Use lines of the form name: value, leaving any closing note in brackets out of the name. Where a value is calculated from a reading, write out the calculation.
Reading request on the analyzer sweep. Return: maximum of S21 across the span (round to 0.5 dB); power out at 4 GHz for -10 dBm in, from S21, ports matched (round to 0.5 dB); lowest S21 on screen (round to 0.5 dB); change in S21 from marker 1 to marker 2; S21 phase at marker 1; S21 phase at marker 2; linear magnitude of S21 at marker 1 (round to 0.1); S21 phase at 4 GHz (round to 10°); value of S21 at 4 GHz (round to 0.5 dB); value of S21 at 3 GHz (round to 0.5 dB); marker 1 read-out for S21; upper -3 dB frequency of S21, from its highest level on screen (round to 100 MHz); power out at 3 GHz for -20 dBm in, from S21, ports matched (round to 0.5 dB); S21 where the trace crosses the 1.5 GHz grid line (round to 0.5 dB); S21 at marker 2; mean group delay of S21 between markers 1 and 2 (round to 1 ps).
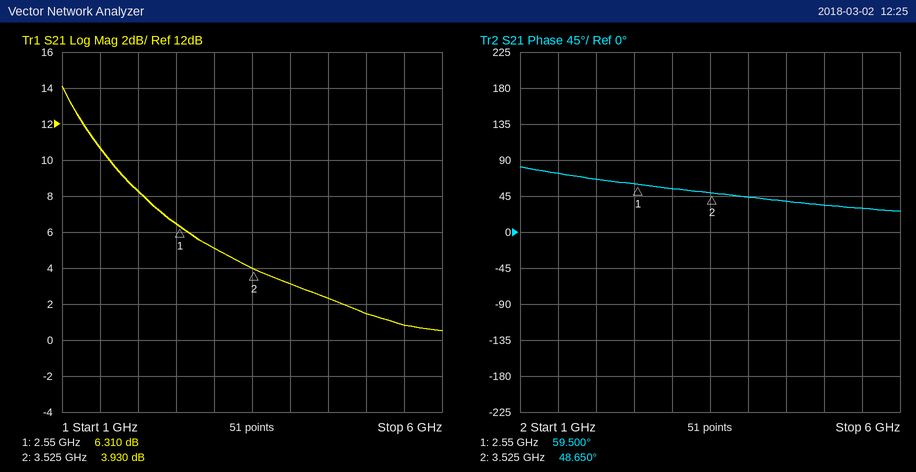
maximum of S21 across the span: 14.0 dB
power out at 4 GHz for -10 dBm in, from S21, ports matched: -10 dBm + (3.0 dB) = -7.0 dBm
lowest S21 on screen: 0.5 dB
change in S21 from marker 1 to marker 2: 3.93 − (6.31) = -2.380 dB
S21 phase at marker 1: 59.500°
S21 phase at marker 2: 48.650°
linear magnitude of S21 at marker 1: 10^(6.31/20) ≈ 2.1
S21 phase at 4 GHz: 40°
value of S21 at 4 GHz: 3.0 dB
value of S21 at 3 GHz: 5.0 dB
marker 1 read-out for S21: 6.310 dB
upper -3 dB frequency of S21, from its highest level on screen: 1.4 GHz
power out at 3 GHz for -20 dBm in, from S21, ports matched: -20 dBm + (5.0 dB) = -15.0 dBm
S21 where the trace crosses the 1.5 GHz grid line: 10.5 dB
S21 at marker 2: 3.930 dB
mean group delay of S21 between markers 1 and 2: −(48.65° − (59.5°))/(360° × 975 MHz) ≈ 31 ps
